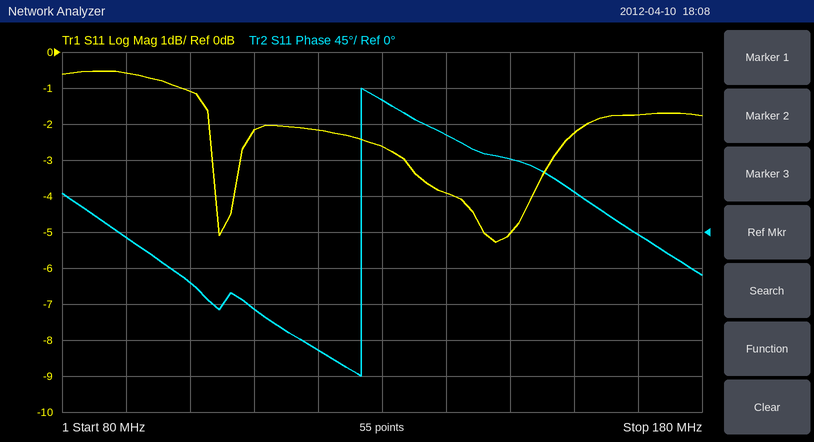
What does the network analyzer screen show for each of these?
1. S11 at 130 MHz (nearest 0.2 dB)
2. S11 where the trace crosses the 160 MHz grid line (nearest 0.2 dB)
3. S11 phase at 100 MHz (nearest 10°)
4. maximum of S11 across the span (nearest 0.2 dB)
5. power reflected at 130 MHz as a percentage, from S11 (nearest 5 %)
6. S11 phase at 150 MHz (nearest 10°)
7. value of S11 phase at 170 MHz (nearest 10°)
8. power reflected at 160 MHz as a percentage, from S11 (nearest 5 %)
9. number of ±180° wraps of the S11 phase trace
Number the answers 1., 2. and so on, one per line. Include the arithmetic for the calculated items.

1. -2.6 dB
2. -2.2 dB
3. -60°
4. -0.6 dB
5. 10^(-2.6/10) ≈ 55 %
6. 90°
7. 0°
8. 10^(-2.2/10) ≈ 60 %
9. 1
